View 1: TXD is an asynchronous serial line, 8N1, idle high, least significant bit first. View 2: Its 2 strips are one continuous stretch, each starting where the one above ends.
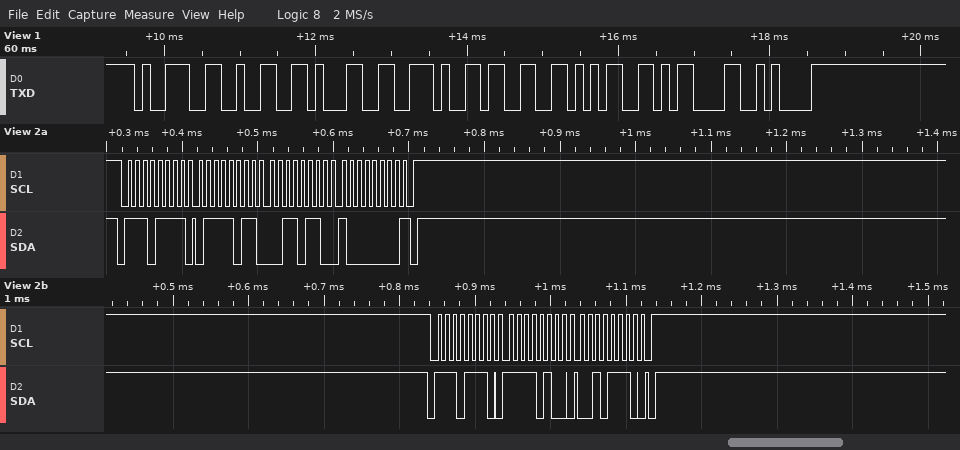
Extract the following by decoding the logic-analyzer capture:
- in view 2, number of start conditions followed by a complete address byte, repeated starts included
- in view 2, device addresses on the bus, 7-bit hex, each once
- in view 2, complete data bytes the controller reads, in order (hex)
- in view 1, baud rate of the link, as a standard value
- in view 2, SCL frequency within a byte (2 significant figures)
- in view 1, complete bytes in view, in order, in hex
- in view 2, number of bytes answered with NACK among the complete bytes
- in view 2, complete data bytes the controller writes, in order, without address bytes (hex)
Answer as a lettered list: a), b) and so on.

a) 2
b) 0x77
c) 7B 36 80
d) 9600 baud
e) 100 kHz
f) 39 32 31 2E 33 35 0D 0A
g) 1
h) F4 2E
